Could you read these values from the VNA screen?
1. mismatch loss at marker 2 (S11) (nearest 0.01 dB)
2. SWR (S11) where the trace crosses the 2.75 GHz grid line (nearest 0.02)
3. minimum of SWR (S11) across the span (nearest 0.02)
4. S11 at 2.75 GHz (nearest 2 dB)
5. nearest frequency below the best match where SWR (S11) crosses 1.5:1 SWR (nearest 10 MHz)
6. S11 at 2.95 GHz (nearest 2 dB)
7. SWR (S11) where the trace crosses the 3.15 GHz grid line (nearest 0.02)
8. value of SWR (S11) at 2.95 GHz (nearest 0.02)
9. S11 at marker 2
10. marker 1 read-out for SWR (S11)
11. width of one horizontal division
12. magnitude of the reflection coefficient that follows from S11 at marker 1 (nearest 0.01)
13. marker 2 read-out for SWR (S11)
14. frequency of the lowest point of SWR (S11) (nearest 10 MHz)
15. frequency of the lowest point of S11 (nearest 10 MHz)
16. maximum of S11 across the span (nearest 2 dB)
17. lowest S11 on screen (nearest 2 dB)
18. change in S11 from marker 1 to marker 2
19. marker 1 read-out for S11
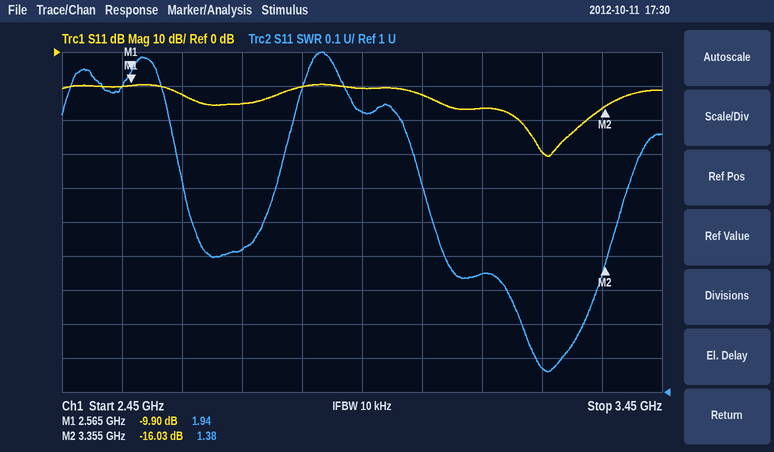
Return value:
0.11 dB
1.42
1.06
-16 dB
3.07 GHz
-10 dB
1.34
1.82
-16.03 dB
1.94
100 MHz
0.32
1.38
3.26 GHz
3.26 GHz
-10 dB
-30 dB
-6.13 dB
-9.90 dB
